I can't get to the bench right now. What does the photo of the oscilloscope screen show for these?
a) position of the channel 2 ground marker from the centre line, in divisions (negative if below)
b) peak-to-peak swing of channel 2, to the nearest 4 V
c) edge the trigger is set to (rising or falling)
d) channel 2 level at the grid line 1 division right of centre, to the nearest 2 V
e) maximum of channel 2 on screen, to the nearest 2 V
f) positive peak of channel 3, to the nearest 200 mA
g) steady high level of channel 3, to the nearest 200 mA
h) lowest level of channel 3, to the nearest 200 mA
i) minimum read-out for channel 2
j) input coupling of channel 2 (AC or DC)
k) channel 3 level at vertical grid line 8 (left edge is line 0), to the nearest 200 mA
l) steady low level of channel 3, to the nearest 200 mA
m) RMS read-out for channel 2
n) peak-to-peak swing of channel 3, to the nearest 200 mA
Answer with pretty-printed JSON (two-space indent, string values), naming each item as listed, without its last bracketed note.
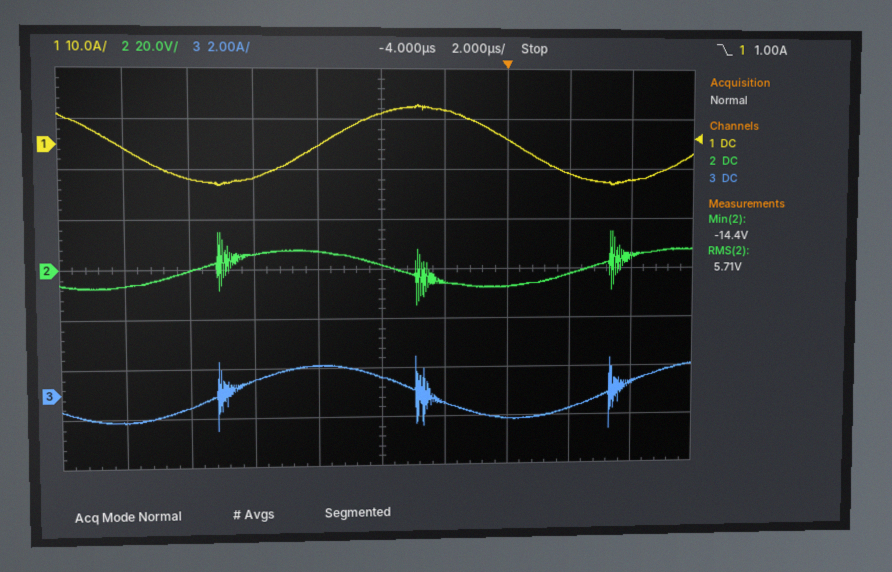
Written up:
{
  "position of the channel 2 ground marker from the centre line, in divisions": "0.0 div",
  "peak-to-peak swing of channel 2, to the nearest 4 V": "28 V",
  "edge the trigger is set to": "falling",
  "channel 2 level at the grid line 1 division right of centre, to the nearest 2 V": "-6 V",
  "maximum of channel 2 on screen, to the nearest 2 V": "16 V",
  "positive peak of channel 3, to the nearest 200 mA": "1.4 A",
  "steady high level of channel 3, to the nearest 200 mA": "1.0 A",
  "lowest level of channel 3, to the nearest 200 mA": "-1.6 A",
  "minimum read-out for channel 2": "-14.4 V",
  "input coupling of channel 2": "DC",
  "channel 3 level at vertical grid line 8 (left edge is line 0), to the nearest 200 mA": "-800 mA",
  "steady low level of channel 3, to the nearest 200 mA": "-1.0 A",
  "RMS read-out for channel 2": "5.71 V",
  "peak-to-peak swing of channel 3, to the nearest 200 mA": "3.0 A"
}
